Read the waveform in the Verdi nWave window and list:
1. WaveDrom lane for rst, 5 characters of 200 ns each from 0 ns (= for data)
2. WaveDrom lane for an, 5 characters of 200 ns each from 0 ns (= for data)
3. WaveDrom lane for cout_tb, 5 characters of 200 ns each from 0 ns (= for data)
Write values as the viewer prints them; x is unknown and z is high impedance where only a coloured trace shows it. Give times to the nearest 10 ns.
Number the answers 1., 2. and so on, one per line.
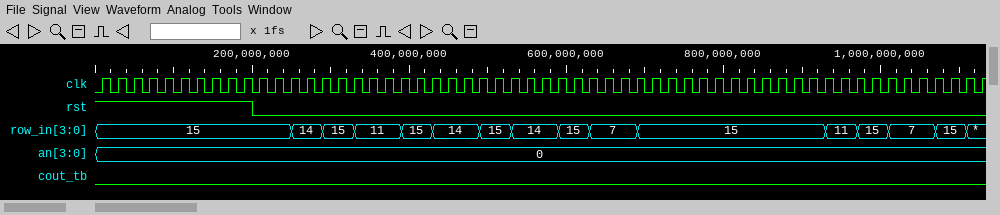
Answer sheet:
1. {name: 'rst', wave: '10...'}
2. {name: 'an', wave: '=....', data: '0'}
3. {name: 'cout_tb', wave: '0....'}
